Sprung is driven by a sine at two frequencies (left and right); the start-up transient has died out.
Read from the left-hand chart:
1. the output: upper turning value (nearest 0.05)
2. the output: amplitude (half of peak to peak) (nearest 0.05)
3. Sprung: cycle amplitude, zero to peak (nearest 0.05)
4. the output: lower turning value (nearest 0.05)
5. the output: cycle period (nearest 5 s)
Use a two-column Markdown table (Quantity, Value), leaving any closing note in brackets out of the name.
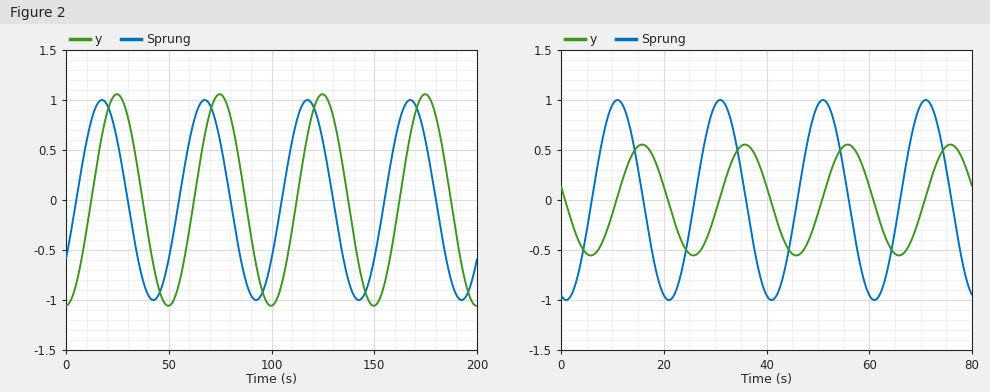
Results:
| Quantity | Value |
|---|---|
| the output: upper turning value | 1.05 |
| the output: amplitude (half of peak to peak) | 1.05 |
| Sprung: cycle amplitude, zero to peak | 1.00 |
| the output: lower turning value | -1.05 |
| the output: cycle period | 50 s |
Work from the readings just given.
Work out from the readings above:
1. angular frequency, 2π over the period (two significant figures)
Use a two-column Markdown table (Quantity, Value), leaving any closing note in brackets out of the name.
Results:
| Quantity | Value |
|---|---|
| angular frequency, 2π over the period | 0.13 rad/s |
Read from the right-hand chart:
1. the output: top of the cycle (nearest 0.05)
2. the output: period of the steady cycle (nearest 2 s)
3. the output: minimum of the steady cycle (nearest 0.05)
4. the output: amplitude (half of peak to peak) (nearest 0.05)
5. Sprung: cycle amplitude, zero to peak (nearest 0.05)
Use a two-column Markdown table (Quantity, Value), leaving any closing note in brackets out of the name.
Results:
| Quantity | Value |
|---|---|
| the output: top of the cycle | 0.55 |
| the output: period of the steady cycle | 20 s |
| the output: minimum of the steady cycle | -0.55 |
| the output: amplitude (half of peak to peak) | 0.55 |
| Sprung: cycle amplitude, zero to peak | 1.00 |
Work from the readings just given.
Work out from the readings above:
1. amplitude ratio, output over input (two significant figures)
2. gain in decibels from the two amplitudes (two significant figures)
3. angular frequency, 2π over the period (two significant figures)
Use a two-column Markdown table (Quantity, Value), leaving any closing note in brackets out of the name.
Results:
| Quantity | Value |
|---|---|
| amplitude ratio, output over input | 0.55 |
| gain in decibels from the two amplitudes | -5.2 dB |
| angular frequency, 2π over the period | 0.31 rad/s |
